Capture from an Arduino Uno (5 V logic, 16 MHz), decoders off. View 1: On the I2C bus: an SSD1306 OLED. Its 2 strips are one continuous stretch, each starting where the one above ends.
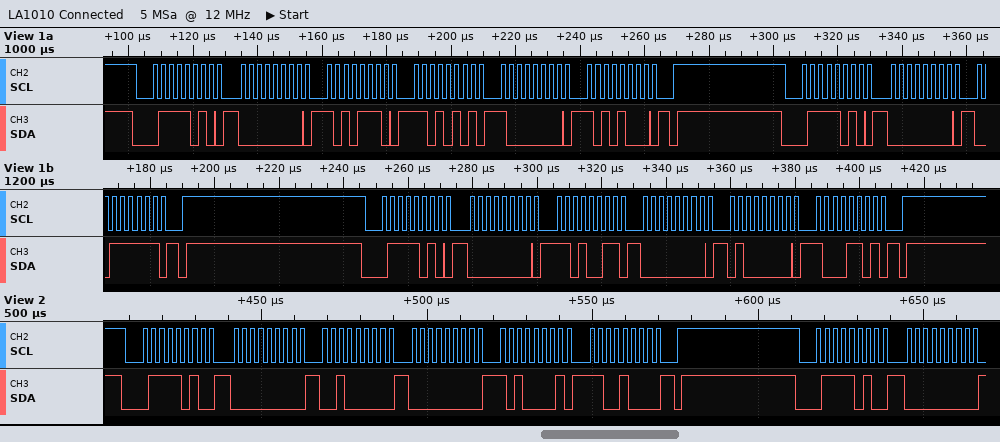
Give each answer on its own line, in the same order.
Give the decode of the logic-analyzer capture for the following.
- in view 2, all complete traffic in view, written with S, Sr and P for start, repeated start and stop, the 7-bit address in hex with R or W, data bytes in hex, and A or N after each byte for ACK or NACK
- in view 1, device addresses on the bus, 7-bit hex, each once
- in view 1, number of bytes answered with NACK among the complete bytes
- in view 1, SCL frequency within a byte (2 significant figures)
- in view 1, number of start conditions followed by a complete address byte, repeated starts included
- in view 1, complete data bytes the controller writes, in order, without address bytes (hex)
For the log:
S 3DW A 00 A 20 A 00 A A1 A C8 A P S 3DW A 00 A
0x3D
0
400 kHz
3
00 AE D5 80 A8 00 3F 00 D3 00 40 8D
